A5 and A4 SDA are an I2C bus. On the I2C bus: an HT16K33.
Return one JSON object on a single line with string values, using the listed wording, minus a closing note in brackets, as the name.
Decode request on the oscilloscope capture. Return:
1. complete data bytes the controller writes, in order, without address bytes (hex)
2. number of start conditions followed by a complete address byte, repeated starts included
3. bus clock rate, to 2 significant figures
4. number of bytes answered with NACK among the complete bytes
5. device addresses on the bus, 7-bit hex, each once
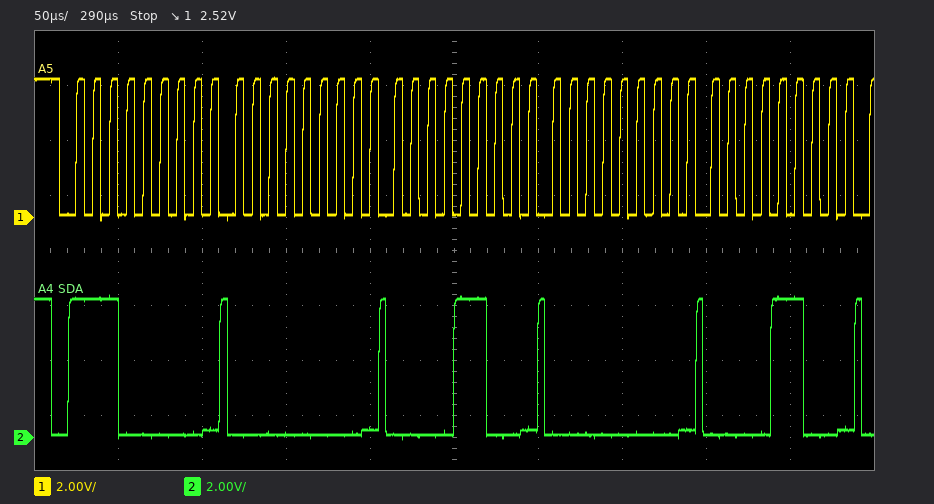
{"complete data bytes the controller writes, in order, without address bytes": "00 0C 00 0C", "number of start conditions followed by a complete address byte, repeated starts included": "1", "bus clock rate, to 2 significant figures": "100 kHz", "number of bytes answered with NACK among the complete bytes": "0", "device addresses on the bus, 7-bit hex, each once": "0x70"}
